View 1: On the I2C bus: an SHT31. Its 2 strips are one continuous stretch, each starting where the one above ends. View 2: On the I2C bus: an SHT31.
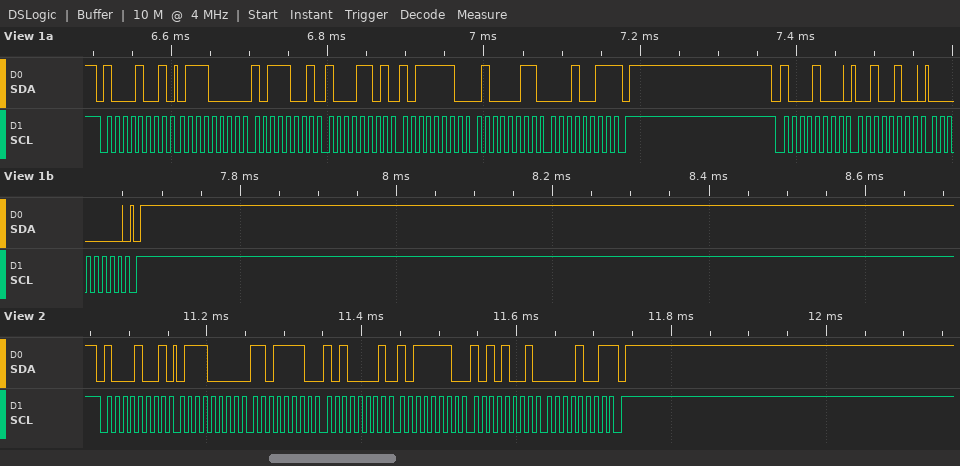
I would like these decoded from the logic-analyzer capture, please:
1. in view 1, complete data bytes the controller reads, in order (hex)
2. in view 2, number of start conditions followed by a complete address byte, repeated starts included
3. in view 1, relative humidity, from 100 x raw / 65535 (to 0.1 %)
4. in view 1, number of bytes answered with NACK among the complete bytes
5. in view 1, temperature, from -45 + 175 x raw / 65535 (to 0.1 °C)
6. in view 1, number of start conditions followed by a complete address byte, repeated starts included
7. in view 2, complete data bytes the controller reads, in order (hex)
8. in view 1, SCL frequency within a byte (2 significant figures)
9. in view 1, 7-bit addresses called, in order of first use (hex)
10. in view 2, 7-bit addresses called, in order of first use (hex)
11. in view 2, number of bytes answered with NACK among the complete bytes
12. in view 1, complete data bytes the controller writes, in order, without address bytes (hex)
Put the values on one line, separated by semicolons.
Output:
70 B9 8D BE 43 13; 1; 74.3 %; 1; 32.1 °C; 2; 70 DE A1 BE A9 09; 100 kHz; 0x44; 0x44; 1; 24 00
